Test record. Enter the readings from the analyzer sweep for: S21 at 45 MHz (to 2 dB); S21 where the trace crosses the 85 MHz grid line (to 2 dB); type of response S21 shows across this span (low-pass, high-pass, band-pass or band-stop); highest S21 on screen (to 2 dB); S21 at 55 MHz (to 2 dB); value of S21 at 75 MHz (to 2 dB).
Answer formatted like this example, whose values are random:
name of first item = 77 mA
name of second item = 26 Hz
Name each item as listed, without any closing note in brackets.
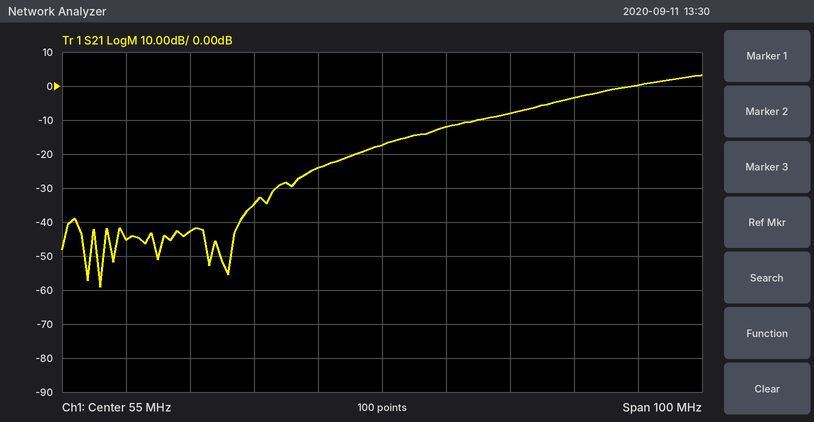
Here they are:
S21 at 45 MHz = -24 dB
S21 where the trace crosses the 85 MHz grid line = -4 dB
type of response S21 shows across this span = high-pass
highest S21 on screen = 4 dB
S21 at 55 MHz = -18 dB
value of S21 at 75 MHz = -8 dB
